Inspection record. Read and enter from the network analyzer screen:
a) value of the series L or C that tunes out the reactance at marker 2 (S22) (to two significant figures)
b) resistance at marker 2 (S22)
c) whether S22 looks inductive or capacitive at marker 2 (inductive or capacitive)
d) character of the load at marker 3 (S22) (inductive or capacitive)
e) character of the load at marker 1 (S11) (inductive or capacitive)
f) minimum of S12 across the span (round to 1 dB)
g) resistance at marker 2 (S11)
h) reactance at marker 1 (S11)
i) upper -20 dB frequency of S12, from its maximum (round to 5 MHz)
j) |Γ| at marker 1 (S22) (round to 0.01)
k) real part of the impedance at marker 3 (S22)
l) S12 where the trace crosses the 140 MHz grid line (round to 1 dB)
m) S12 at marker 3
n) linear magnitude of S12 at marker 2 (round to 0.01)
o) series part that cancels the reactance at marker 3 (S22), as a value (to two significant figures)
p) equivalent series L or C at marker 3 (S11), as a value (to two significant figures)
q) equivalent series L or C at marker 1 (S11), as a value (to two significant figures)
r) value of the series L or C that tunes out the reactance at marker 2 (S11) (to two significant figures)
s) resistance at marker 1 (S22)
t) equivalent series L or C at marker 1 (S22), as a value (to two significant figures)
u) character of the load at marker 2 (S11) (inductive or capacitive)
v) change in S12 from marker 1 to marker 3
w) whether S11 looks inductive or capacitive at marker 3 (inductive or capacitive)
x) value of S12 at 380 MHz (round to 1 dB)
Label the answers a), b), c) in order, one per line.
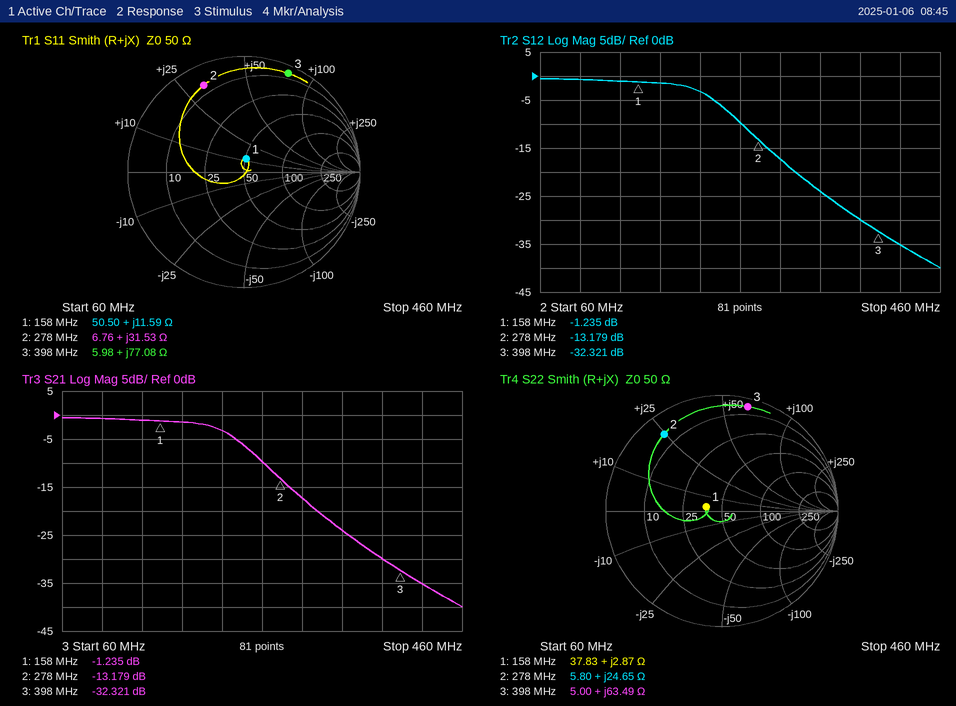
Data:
a) 23 pF
b) 5.80 Ω
c) inductive
d) inductive
e) inductive
f) -40 dB
g) 6.76 Ω
h) +11.59 Ω
i) 320 MHz
j) 0.14
k) 5.00 Ω
l) -1 dB
m) -32.321 dB
n) 0.22
o) 6.3 pF
p) 31 nH
q) 12 nH
r) 18 pF
s) 37.83 Ω
t) 2.9 nH
u) inductive
v) -31.086 dB
w) inductive
x) -30 dB
